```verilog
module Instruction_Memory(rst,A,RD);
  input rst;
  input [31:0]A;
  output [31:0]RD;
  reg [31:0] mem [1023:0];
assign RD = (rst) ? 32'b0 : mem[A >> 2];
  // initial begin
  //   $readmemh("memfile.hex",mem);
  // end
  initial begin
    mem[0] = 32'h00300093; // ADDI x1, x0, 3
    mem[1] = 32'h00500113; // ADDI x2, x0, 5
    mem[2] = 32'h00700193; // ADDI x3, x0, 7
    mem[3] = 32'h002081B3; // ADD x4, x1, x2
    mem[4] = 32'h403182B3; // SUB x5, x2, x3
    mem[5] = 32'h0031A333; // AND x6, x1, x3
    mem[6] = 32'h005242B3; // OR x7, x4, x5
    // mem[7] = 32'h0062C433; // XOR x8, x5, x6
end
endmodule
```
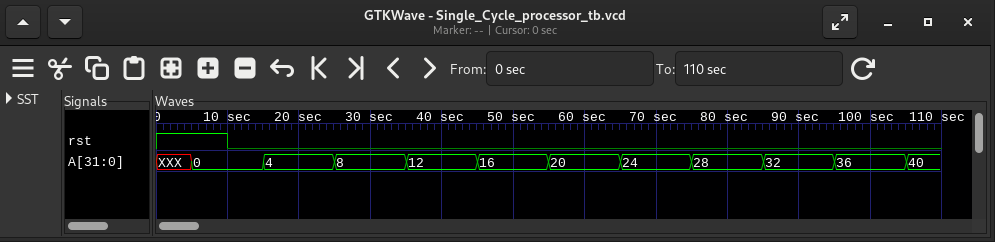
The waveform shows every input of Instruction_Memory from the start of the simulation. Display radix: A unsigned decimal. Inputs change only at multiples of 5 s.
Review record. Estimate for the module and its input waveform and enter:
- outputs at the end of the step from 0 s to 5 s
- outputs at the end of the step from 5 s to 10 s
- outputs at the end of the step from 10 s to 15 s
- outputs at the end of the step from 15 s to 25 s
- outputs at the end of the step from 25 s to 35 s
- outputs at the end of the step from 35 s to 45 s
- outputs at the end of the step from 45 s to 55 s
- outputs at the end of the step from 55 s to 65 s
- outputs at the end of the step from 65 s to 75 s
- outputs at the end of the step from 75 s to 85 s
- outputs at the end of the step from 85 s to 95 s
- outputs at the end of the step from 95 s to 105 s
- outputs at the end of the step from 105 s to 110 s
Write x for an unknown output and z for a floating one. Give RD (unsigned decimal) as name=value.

RD=0
RD=0
RD=3145875
RD=5243155
RD=7340435
RD=2130355
RD=1076986547
RD=3253043
RD=5391027
RD=x
RD=x
RD=x
RD=x
